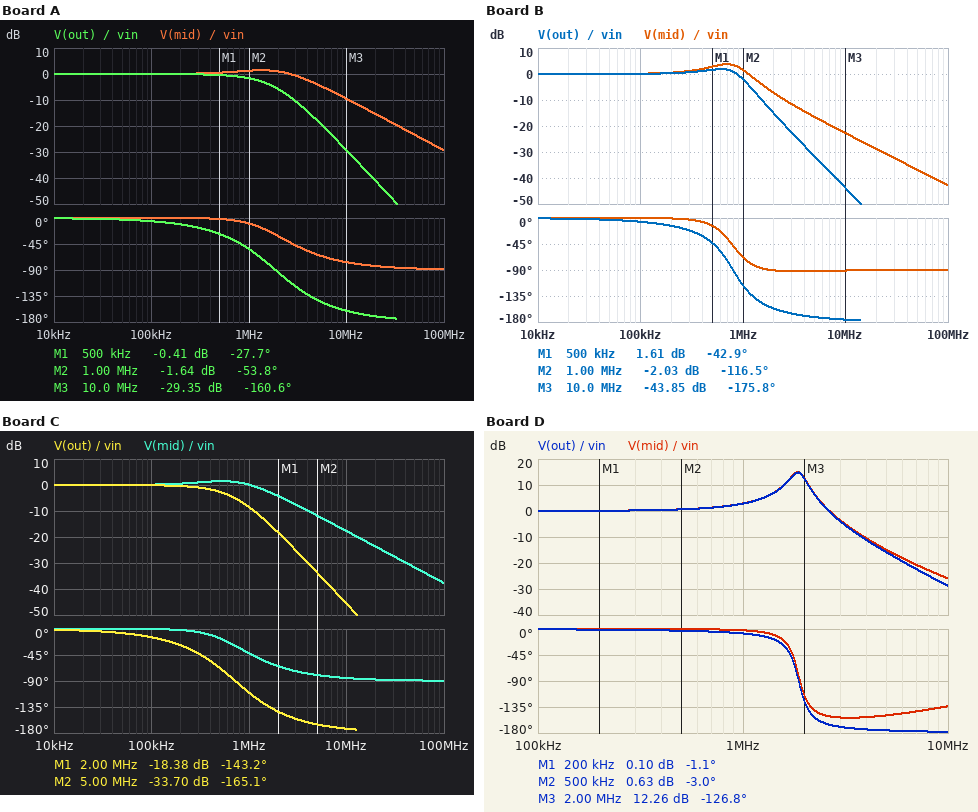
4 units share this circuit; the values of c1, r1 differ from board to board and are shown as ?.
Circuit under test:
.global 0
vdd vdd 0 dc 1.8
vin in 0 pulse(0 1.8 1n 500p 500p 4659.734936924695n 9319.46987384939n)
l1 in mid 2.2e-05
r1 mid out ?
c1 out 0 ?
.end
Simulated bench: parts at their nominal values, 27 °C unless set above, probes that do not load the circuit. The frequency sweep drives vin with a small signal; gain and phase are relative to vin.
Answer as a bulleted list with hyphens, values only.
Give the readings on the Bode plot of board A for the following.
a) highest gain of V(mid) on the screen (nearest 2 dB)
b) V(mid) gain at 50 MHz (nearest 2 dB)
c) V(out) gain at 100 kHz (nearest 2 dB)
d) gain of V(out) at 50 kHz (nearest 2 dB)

- 2 dB
- -24 dB
- 0 dB
- 0 dB
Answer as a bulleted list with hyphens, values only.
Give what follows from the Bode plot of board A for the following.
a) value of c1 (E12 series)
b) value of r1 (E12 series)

- 330 pF
- 470 Ω
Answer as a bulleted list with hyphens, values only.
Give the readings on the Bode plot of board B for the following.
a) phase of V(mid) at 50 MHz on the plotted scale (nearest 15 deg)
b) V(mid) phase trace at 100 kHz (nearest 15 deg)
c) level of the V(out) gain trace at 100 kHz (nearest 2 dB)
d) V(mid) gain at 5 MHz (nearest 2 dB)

- -90 deg
- 0 deg
- 0 dB
- -16 dB
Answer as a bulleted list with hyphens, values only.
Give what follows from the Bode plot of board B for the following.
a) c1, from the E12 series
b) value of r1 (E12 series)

- 1.8 nF
- 100 Ω
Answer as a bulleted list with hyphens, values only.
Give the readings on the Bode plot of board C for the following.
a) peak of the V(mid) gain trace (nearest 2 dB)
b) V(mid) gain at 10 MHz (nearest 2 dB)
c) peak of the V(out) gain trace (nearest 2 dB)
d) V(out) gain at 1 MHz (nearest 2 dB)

- 2 dB
- -18 dB
- 0 dB
- -8 dB
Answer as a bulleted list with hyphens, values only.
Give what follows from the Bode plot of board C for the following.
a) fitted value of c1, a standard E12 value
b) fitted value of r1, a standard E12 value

- 2.2 nF
- 180 Ω
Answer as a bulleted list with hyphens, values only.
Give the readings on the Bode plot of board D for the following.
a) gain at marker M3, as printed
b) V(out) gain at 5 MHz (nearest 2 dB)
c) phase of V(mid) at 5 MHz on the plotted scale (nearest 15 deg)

- 12.26 dB
- -16 dB
- -150 deg
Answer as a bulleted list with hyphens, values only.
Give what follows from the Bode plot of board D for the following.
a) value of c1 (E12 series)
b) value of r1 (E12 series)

- 330 pF
- 47 Ω
